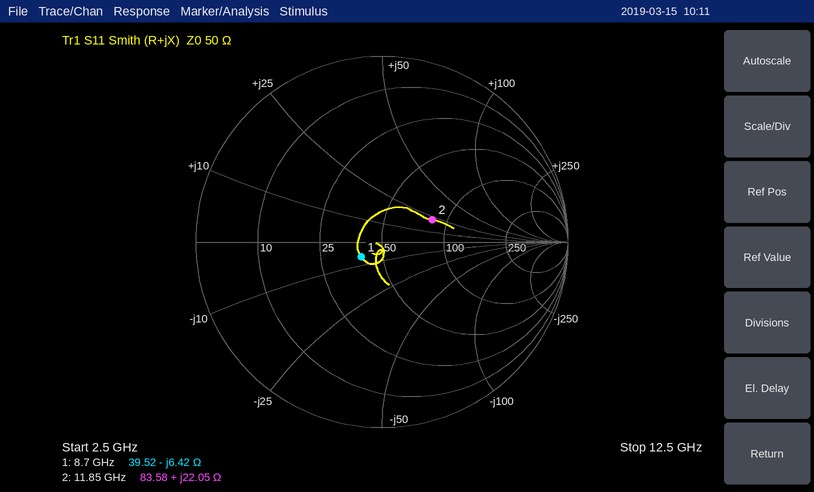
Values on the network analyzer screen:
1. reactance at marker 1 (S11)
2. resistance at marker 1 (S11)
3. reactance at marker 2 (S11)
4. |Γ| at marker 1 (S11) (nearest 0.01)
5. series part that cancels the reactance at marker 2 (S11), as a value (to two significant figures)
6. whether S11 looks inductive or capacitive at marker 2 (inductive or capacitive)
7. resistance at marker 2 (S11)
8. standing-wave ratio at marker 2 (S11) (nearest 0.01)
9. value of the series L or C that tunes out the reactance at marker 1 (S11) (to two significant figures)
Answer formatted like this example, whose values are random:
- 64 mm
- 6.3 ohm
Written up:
- -6.42 Ω
- 39.52 Ω
- +22.05 Ω
- 0.14
- 610 fF
- inductive
- 83.58 Ω
- 1.84
- 120 pH
